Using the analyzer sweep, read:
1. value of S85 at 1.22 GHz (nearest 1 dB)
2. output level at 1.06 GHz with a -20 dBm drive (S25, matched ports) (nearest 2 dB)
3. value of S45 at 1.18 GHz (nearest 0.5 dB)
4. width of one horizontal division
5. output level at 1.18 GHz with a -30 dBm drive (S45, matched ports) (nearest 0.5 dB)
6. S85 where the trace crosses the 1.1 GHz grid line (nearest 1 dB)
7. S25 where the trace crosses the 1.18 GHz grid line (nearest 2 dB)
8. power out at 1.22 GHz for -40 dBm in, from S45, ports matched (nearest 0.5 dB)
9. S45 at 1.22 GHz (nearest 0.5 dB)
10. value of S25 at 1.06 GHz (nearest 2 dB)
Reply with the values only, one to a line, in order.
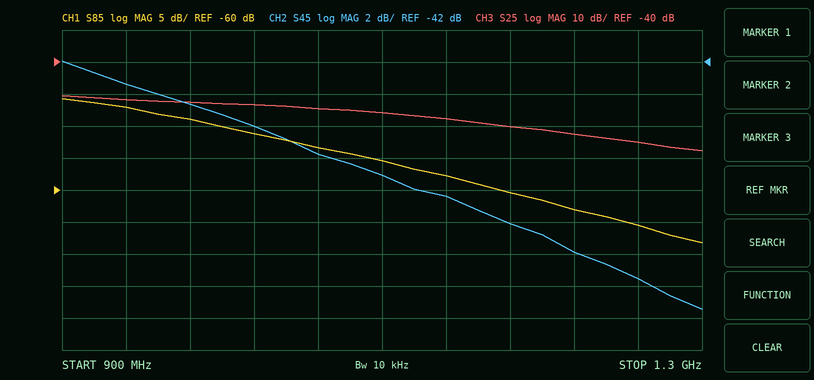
-63 dB
-74 dBm
-52.0 dB
40 MHz
-82.0 dBm
-55 dB
-60 dB
-94.0 dBm
-54.0 dB
-54 dB
